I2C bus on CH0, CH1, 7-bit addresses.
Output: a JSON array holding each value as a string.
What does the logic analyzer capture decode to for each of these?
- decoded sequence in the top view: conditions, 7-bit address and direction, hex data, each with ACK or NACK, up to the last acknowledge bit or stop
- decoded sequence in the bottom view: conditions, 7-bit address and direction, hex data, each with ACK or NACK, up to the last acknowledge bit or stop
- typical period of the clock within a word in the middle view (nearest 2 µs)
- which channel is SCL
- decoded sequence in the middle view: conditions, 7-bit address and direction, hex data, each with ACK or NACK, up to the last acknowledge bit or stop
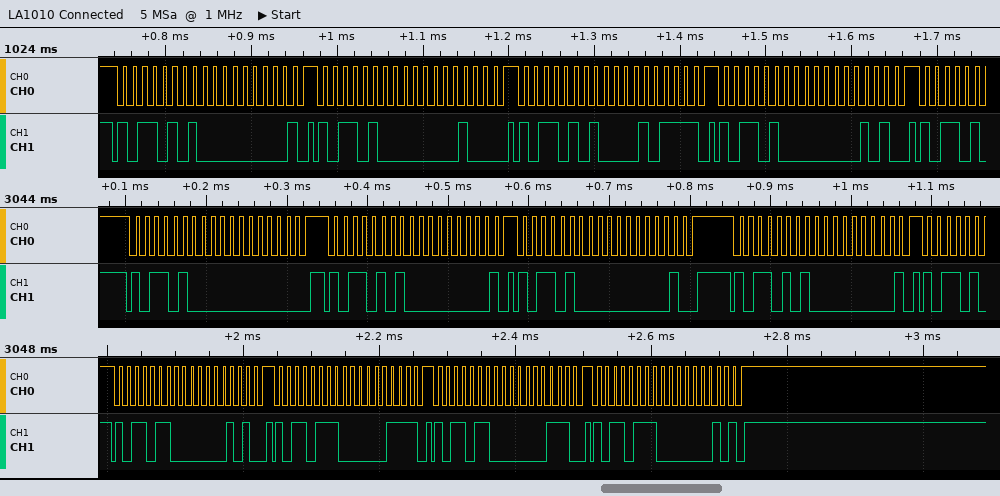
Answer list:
["start, address 5A read ACK, 00 NACK, stop, start, address 5A write ACK, 04 ACK, stop, start, address 5A read ACK, 17 NACK, stop, start, address 5A write ACK, 05 ACK, stop", "start, address 5B write ACK, 05 ACK, stop, start, address 5B read ACK, 07 NACK, stop, start, address 5B write ACK, 07 ACK, stop, start, address 5B read ACK, 02 NACK, stop", "12 µs", "CH0", "start, address 5A write ACK, 00 ACK, stop, start, address 5A read ACK, 00 NACK, stop, start, address 5A write ACK, 01 ACK, stop, start, address 5A read ACK, 00 NACK, stop"]
